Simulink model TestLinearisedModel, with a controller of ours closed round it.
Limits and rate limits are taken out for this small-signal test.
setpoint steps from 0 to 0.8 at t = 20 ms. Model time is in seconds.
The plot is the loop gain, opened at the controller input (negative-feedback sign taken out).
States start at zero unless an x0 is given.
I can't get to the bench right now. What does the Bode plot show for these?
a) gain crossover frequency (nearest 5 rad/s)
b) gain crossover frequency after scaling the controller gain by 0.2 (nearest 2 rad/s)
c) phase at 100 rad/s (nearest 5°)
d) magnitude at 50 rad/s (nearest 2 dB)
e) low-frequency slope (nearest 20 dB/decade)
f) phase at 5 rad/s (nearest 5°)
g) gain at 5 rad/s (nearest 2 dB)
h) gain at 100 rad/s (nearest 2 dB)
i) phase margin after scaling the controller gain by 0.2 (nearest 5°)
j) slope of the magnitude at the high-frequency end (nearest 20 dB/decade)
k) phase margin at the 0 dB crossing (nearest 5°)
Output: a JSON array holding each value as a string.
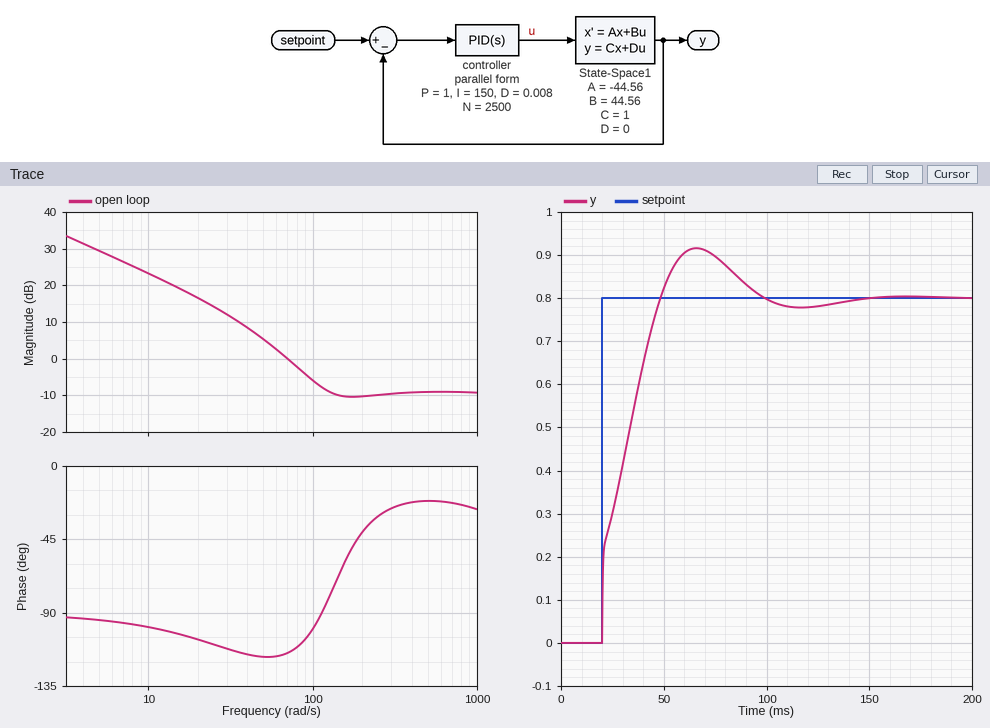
["70 rad/s", "26 rad/s", "-100°", "6 dB", "-20 dB/decade", "-95°", "30 dB", "-6 dB", "70°", "0 dB/decade", "65°"]
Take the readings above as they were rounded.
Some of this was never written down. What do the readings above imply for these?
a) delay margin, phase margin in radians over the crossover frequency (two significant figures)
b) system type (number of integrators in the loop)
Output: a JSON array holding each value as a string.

["0.016 s", "1"]
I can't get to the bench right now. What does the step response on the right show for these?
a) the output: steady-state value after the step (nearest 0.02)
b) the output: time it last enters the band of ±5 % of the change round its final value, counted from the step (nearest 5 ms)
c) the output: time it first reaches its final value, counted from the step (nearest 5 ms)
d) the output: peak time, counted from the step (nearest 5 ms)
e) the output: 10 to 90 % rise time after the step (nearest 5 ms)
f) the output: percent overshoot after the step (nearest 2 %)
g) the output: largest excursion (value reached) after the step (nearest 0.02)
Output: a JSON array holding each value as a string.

["0.80", "70 ms", "30 ms", "45 ms", "25 ms", "14 %", "0.92"]
